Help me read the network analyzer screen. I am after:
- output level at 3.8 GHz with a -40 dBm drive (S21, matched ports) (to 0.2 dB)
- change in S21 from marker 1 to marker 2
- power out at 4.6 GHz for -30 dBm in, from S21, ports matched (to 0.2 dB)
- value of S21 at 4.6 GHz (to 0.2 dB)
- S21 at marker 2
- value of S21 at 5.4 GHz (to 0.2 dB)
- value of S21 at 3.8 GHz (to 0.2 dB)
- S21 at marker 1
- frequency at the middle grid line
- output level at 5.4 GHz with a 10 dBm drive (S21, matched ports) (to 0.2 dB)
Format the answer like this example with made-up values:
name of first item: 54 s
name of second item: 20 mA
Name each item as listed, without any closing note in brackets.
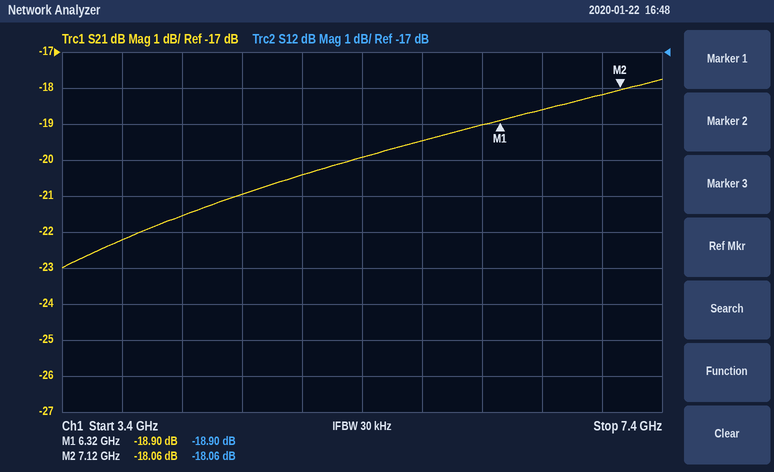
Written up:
output level at 3.8 GHz with a -40 dBm drive (S21, matched ports): -62.2 dBm
change in S21 from marker 1 to marker 2: 0.84 dB
power out at 4.6 GHz for -30 dBm in, from S21, ports matched: -51.0 dBm
value of S21 at 4.6 GHz: -21.0 dB
S21 at marker 2: -18.06 dB
value of S21 at 5.4 GHz: -20.0 dB
value of S21 at 3.8 GHz: -22.2 dB
S21 at marker 1: -18.90 dB
frequency at the middle grid line: 5.4 GHz
output level at 5.4 GHz with a 10 dBm drive (S21, matched ports): -10.0 dBm
